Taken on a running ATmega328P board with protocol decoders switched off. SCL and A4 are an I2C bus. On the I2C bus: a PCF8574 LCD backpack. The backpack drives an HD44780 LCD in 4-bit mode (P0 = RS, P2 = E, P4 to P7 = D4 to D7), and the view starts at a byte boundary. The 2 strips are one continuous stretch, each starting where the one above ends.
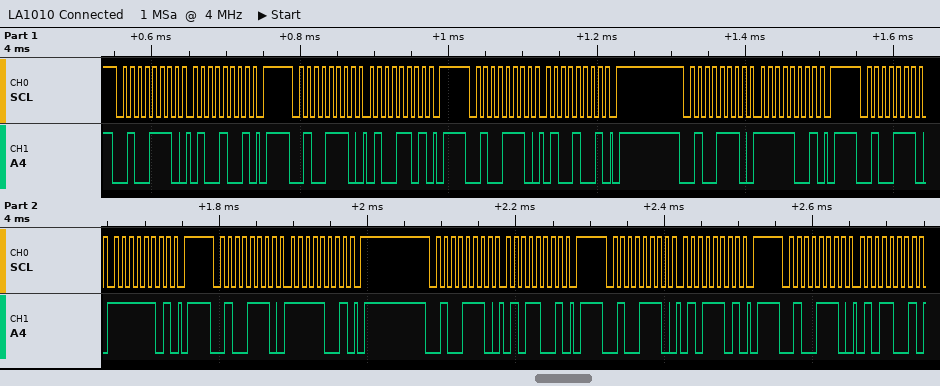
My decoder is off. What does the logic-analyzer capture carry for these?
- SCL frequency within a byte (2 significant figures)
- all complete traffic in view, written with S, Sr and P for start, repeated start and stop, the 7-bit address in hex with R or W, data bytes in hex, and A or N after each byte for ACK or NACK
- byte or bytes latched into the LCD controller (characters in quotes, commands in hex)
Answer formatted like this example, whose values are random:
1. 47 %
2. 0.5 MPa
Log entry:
1. 100 kHz
2. S 27W A 49 A P S 27W A 4D A P S 27W A 49 A P S 27W A F9 A P S 27W A FD A P S 27W A F9 A P S 27W A 59 A P S 27W A 5D A P S 27W A 59 A
3. 'O'
